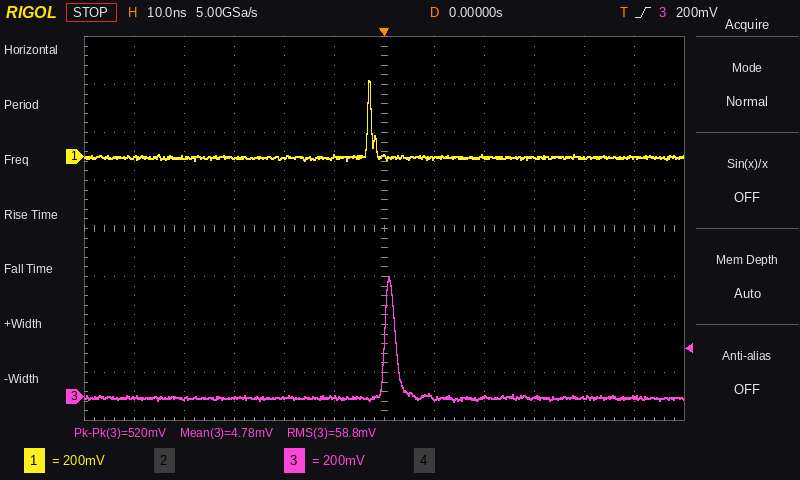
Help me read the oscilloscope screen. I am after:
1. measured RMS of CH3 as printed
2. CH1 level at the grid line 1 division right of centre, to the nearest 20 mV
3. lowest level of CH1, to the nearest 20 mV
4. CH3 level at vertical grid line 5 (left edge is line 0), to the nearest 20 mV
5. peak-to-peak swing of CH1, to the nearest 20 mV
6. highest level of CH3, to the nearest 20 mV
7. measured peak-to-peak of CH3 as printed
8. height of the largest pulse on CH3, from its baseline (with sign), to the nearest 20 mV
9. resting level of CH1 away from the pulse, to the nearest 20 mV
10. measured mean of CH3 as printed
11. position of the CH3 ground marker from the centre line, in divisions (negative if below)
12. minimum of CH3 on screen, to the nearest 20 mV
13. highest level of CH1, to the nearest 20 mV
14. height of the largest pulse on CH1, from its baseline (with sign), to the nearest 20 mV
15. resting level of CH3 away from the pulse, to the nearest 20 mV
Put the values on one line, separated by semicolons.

58.8 mV; 0 mV; -20 mV; 0 mV; 340 mV; 500 mV; 520 mV; +500 mV; 0 mV; 4.78 mV; -3.5 div; -20 mV; 320 mV; +320 mV; 0 mV
